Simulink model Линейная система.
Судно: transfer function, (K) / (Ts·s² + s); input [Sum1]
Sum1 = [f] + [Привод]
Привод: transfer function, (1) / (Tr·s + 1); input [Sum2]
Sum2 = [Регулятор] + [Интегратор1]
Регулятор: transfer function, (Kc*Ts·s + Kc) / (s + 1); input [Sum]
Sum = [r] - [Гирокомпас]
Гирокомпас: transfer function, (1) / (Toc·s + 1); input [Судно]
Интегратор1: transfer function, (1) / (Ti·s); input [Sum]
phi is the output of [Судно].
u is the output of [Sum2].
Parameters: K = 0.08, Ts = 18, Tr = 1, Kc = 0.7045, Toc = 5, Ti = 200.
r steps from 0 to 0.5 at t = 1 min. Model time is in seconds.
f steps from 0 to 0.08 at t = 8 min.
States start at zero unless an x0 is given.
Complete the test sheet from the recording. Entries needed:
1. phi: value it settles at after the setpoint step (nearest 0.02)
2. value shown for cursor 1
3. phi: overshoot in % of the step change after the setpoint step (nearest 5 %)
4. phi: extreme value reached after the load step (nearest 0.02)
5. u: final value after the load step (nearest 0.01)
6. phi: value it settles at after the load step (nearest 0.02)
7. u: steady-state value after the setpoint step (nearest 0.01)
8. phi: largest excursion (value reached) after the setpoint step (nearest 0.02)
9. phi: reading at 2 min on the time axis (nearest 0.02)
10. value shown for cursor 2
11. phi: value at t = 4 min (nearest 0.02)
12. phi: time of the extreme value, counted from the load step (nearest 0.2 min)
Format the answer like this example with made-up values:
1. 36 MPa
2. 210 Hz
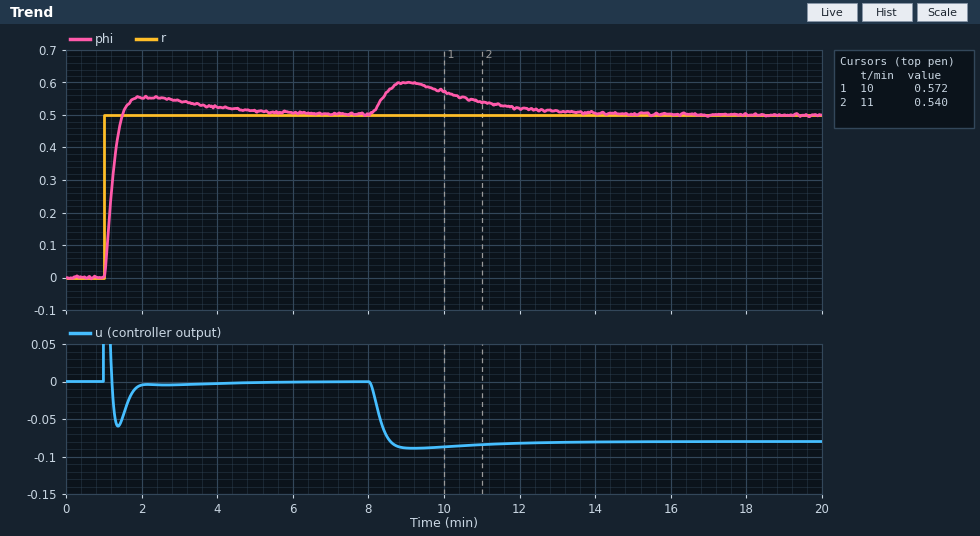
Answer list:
1. 0.50
2. 0.572
3. 10 %
4. 0.60
5. -0.08
6. 0.50
7. 0.00
8. 0.56
9. 0.56
10. 0.540
11. 0.52
12. 1.0 min
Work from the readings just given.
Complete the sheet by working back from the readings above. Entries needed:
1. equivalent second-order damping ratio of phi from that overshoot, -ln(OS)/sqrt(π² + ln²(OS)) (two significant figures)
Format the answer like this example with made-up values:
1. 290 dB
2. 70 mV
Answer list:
1. 0.59
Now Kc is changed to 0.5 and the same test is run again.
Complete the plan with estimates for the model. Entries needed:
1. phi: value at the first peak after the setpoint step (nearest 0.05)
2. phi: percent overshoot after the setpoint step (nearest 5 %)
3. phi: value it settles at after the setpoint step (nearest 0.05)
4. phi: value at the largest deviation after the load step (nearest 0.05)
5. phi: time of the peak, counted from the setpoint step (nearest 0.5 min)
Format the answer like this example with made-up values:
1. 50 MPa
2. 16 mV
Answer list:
1. 0.60
2. 20 %
3. 0.50
4. 0.65
5. 1.5 min
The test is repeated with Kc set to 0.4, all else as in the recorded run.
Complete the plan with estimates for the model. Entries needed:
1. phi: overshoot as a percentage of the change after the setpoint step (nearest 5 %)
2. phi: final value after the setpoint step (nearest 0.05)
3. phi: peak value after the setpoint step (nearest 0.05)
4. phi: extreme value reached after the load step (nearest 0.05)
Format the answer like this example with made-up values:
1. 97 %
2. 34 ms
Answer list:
1. 25 %
2. 0.50
3. 0.65
4. 0.65
